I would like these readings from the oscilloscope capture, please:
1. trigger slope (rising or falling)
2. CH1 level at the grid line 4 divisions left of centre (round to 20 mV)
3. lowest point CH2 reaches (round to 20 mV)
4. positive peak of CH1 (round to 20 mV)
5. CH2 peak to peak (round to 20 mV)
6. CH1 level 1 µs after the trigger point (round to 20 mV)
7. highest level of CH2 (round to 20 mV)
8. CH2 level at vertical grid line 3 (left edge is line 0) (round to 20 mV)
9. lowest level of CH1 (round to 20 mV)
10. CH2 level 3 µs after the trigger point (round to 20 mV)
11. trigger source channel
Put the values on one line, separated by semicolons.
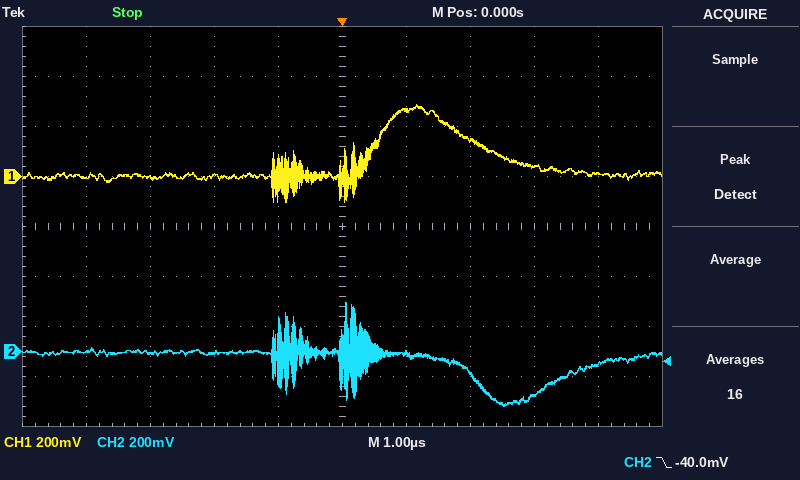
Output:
falling; 0 mV; -220 mV; 280 mV; 420 mV; 260 mV; 200 mV; 0 mV; -100 mV; -180 mV; CH2
